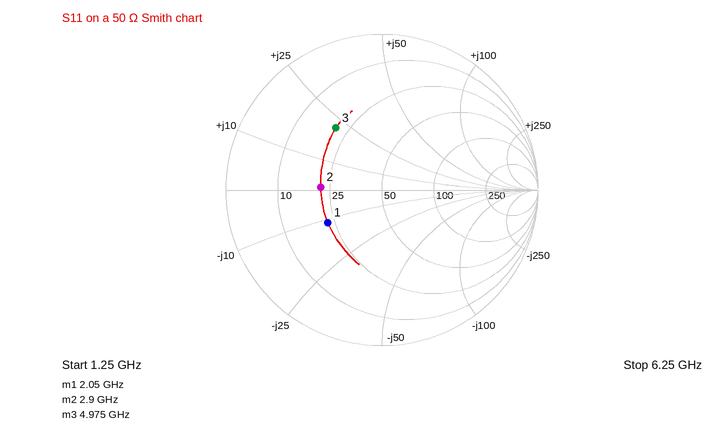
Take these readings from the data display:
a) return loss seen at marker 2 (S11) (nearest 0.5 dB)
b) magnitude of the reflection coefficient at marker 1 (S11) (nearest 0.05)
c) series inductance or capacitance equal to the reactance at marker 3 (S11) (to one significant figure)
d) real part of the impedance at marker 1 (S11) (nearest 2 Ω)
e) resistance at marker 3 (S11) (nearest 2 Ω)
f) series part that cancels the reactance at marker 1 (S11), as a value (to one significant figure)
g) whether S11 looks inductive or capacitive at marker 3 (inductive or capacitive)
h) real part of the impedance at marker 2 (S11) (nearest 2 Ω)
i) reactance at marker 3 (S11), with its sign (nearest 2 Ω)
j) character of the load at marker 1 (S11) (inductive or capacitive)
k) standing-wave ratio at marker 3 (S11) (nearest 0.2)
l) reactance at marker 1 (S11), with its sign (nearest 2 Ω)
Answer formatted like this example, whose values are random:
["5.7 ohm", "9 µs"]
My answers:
["8.0 dB", "0.40", "700 pH", "22 Ω", "20 Ω", "900 pH", "inductive", "22 Ω", "+22 Ω", "capacitive", "3.0", "-12 Ω"]
